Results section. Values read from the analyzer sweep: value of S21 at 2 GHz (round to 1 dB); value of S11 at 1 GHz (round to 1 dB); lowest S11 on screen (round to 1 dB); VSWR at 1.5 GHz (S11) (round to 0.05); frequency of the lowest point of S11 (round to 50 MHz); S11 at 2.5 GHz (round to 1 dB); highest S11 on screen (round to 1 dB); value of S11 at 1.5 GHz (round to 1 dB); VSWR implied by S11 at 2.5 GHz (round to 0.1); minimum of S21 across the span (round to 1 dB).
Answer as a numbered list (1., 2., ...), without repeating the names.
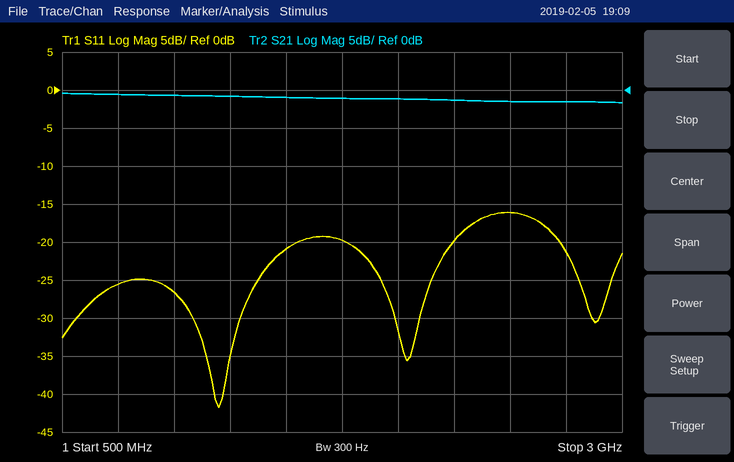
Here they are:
1. -1 dB
2. -27 dB
3. -42 dB
4. 1.20
5. 1.20 GHz
6. -16 dB
7. -16 dB
8. -21 dB
9. 1.4
10. -2 dB
